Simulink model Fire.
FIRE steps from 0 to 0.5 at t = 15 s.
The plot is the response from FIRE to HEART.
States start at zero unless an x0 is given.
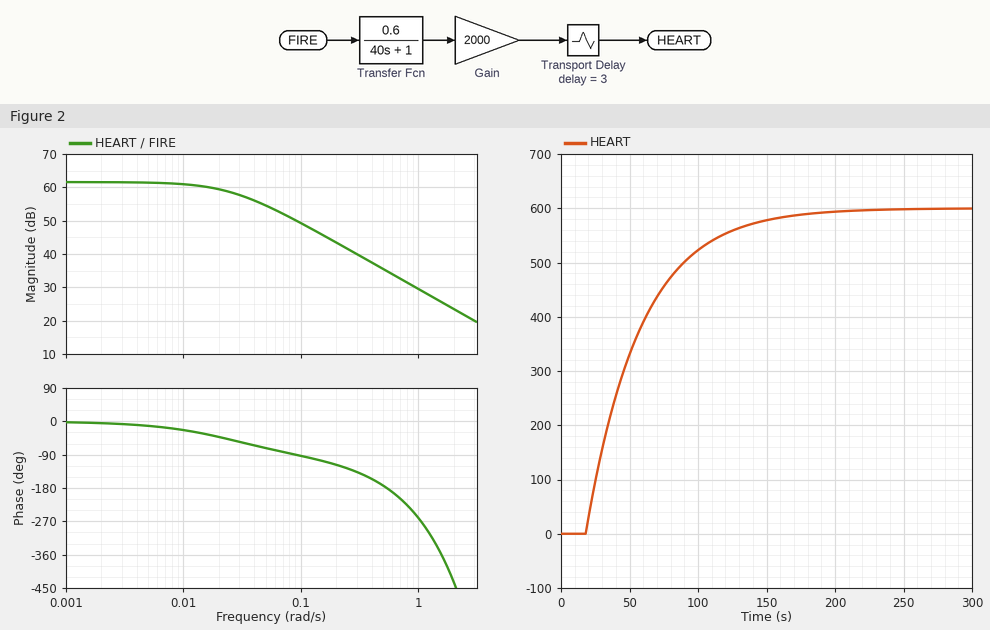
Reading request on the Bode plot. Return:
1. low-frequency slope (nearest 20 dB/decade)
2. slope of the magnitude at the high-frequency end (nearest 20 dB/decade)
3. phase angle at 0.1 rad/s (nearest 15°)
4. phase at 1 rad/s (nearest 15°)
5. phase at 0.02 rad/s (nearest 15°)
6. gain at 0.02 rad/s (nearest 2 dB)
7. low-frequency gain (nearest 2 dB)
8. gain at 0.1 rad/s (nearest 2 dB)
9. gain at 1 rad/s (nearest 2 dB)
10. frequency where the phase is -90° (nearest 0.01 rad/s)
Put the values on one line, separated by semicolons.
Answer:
0 dB/decade; -20 dB/decade; -90°; -255°; -45°; 60 dB; 62 dB; 50 dB; 30 dB; 0.09 rad/s
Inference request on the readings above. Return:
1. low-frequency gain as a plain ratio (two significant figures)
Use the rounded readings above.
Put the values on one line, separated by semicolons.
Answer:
1300
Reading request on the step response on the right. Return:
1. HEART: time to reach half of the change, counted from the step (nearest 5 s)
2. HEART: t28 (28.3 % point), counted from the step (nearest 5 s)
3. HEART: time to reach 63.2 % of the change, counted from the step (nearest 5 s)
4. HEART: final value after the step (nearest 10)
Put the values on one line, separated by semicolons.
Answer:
30 s; 15 s; 45 s; 600
